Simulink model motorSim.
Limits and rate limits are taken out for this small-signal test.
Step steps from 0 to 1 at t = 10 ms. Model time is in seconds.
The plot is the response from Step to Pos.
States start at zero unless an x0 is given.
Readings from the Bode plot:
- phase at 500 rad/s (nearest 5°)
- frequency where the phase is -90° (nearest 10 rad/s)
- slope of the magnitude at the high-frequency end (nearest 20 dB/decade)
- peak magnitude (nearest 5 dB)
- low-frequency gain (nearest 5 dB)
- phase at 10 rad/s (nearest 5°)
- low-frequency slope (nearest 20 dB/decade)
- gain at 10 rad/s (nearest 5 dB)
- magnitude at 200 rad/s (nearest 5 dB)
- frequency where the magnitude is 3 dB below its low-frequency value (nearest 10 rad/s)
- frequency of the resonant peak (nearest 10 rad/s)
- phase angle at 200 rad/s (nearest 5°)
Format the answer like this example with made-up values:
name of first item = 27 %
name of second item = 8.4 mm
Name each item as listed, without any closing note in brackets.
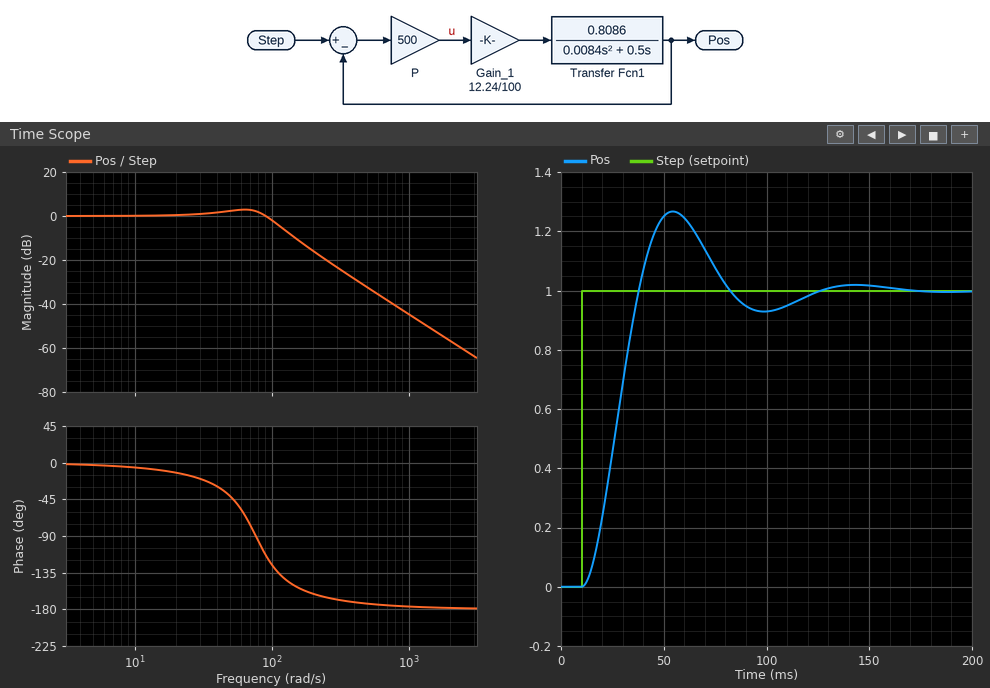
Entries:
phase at 500 rad/s = -175°
frequency where the phase is -90° = 80 rad/s
slope of the magnitude at the high-frequency end = -40 dB/decade
peak magnitude = 5 dB
low-frequency gain = 0 dB
phase at 10 rad/s = -5°
low-frequency slope = 0 dB/decade
gain at 10 rad/s = 0 dB
magnitude at 200 rad/s = -15 dB
frequency where the magnitude is 3 dB below its low-frequency value = 110 rad/s
frequency of the resonant peak = 60 rad/s
phase angle at 200 rad/s = -160°
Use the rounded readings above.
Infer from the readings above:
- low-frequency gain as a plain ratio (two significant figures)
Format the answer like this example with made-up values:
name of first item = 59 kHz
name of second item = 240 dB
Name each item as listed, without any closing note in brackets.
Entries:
low-frequency gain as a plain ratio = 1.0
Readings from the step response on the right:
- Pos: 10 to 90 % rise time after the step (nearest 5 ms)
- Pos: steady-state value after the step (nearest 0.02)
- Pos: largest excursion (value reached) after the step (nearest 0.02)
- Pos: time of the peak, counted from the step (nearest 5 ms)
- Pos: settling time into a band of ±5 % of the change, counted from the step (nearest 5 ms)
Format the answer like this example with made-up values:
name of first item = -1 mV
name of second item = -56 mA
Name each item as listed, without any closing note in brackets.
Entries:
Pos: 10 to 90 % rise time after the step = 20 ms
Pos: steady-state value after the step = 1.00
Pos: largest excursion (value reached) after the step = 1.26
Pos: time of the peak, counted from the step = 45 ms
Pos: settling time into a band of ±5 % of the change, counted from the step = 100 ms
